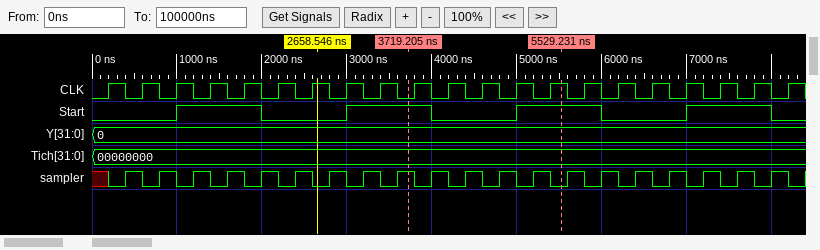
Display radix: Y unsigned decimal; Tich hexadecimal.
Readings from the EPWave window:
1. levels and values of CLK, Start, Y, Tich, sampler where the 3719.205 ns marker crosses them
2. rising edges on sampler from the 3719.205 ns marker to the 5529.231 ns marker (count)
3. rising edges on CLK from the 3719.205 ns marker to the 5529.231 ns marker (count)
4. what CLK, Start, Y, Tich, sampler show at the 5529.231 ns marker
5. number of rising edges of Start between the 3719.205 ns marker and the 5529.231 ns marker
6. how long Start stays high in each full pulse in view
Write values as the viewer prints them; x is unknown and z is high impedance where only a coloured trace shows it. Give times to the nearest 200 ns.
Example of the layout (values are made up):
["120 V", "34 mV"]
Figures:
["CLK=0, Start=1, Y=0, Tich=00000000, sampler=1", "4", "5", "CLK=1, Start=1, Y=0, Tich=00000000, sampler=0", "1", "1000 ns, 1000 ns, 1000 ns, 1000 ns"]
